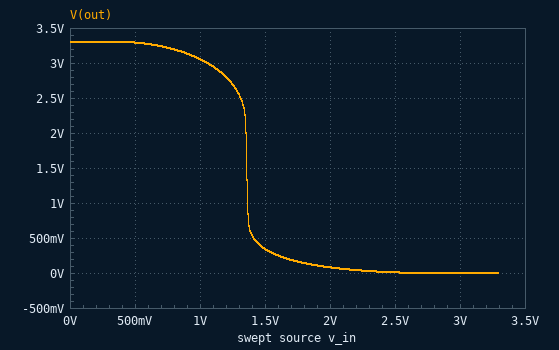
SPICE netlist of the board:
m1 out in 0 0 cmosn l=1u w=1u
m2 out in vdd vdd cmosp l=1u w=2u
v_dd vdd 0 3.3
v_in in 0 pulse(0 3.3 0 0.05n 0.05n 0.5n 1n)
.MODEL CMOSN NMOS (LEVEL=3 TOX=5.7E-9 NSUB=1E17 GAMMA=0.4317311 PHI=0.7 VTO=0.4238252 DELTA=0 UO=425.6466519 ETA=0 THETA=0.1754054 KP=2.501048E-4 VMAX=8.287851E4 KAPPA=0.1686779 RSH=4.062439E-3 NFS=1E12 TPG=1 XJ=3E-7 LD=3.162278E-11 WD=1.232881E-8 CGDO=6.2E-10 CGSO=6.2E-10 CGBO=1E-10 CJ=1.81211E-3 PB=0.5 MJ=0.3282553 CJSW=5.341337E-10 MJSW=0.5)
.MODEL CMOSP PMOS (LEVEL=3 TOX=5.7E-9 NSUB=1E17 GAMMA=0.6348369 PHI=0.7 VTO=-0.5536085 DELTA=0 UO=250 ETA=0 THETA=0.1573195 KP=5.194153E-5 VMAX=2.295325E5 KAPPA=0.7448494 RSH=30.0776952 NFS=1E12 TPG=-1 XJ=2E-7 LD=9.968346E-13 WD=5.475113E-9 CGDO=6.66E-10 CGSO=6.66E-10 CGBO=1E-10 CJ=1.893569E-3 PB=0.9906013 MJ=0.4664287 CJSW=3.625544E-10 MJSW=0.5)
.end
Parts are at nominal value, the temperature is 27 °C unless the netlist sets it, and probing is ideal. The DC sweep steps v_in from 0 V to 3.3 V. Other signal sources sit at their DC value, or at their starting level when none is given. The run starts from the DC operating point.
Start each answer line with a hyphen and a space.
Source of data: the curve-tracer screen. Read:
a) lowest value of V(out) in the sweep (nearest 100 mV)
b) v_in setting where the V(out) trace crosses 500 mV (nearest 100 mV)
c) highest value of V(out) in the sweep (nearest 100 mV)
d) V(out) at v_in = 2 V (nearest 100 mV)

- 0 V
- 1.4 V
- 3.3 V
- 100 mV
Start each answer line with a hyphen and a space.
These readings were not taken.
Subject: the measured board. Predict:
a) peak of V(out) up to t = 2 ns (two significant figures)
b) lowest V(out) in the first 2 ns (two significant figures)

- 3.9 V
- -610 mV
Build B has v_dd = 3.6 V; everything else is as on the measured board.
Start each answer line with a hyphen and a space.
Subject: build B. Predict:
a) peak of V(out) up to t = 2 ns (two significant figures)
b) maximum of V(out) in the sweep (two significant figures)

- 4.2 V
- 3.6 V
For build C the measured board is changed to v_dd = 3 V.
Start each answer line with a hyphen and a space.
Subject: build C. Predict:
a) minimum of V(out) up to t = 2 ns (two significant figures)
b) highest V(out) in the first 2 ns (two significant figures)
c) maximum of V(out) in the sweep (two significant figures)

- -620 mV
- 3.6 V
- 3.0 V
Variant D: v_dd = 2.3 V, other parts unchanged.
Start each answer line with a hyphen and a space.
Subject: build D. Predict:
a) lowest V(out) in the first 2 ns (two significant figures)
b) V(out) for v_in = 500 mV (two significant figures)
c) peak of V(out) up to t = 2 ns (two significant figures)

- -620 mV
- 2.3 V
- 2.9 V
